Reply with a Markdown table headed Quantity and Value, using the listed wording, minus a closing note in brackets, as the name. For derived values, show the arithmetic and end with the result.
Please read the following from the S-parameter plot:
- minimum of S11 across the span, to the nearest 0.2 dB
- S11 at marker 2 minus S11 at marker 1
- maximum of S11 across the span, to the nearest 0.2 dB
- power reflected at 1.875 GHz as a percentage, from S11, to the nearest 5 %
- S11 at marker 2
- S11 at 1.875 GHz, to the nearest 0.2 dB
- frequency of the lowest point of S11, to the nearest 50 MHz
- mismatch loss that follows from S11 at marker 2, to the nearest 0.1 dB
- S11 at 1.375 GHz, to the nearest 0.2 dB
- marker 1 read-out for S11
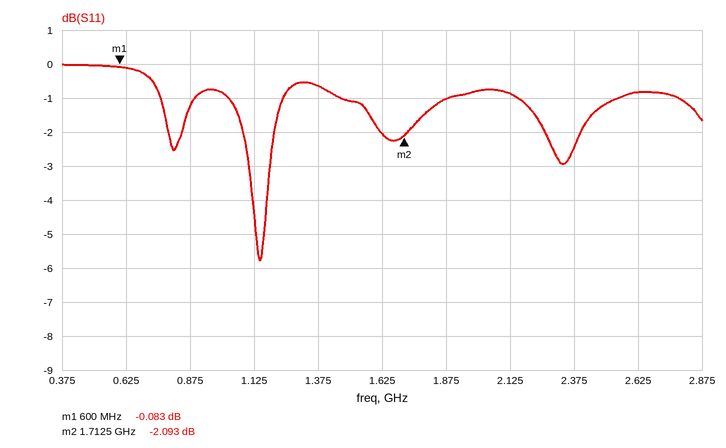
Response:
| Quantity | Value |
|---|---|
| minimum of S11 across the span, to the nearest 0.2 dB | -5.8 dB |
| S11 at marker 2 minus S11 at marker 1 | -2.093 − (-0.083) = -2.010 dB |
| maximum of S11 across the span, to the nearest 0.2 dB | 0.0 dB |
| power reflected at 1.875 GHz as a percentage, from S11, to the nearest 5 % | 10^(-1/10) ≈ 79.4 %, so 80 % to the nearest 5 % |
| S11 at marker 2 | -2.093 dB |
| S11 at 1.875 GHz, to the nearest 0.2 dB | -1.0 dB |
| frequency of the lowest point of S11, to the nearest 50 MHz | 1.15 GHz |
| mismatch loss that follows from S11 at marker 2, to the nearest 0.1 dB | −10 log10(1 − 10^(-2.093/10)) ≈ 4.2 dB |
| S11 at 1.375 GHz, to the nearest 0.2 dB | -0.6 dB |
| marker 1 read-out for S11 | -0.083 dB |
